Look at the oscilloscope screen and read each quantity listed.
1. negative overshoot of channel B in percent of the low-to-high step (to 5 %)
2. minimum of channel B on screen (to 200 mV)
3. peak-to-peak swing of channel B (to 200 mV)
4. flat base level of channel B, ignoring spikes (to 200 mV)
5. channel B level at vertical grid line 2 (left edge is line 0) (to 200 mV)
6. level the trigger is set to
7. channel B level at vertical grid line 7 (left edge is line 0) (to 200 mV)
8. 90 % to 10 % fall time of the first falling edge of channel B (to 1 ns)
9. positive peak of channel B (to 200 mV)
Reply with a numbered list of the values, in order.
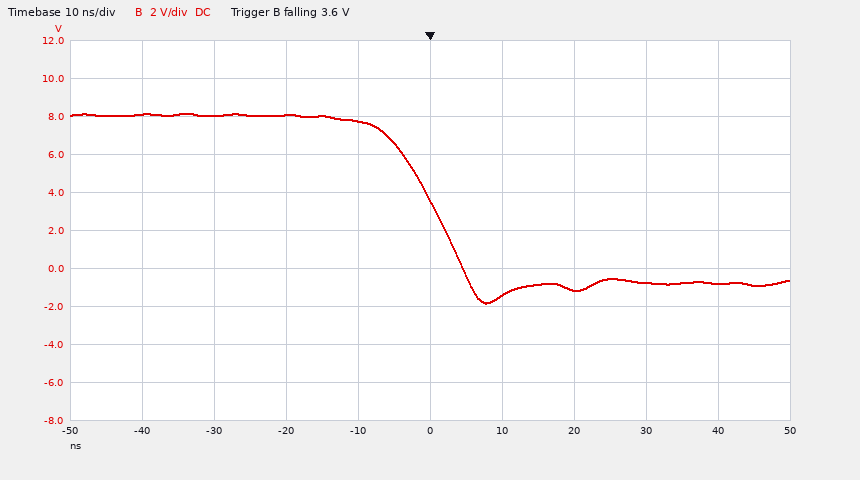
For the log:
1. 10 %
2. -1.8 V
3. 10.0 V
4. -800 mV
5. 8.0 V
6. 3.6 V
7. -1.2 V
8. 11 ns
9. 8.2 V
